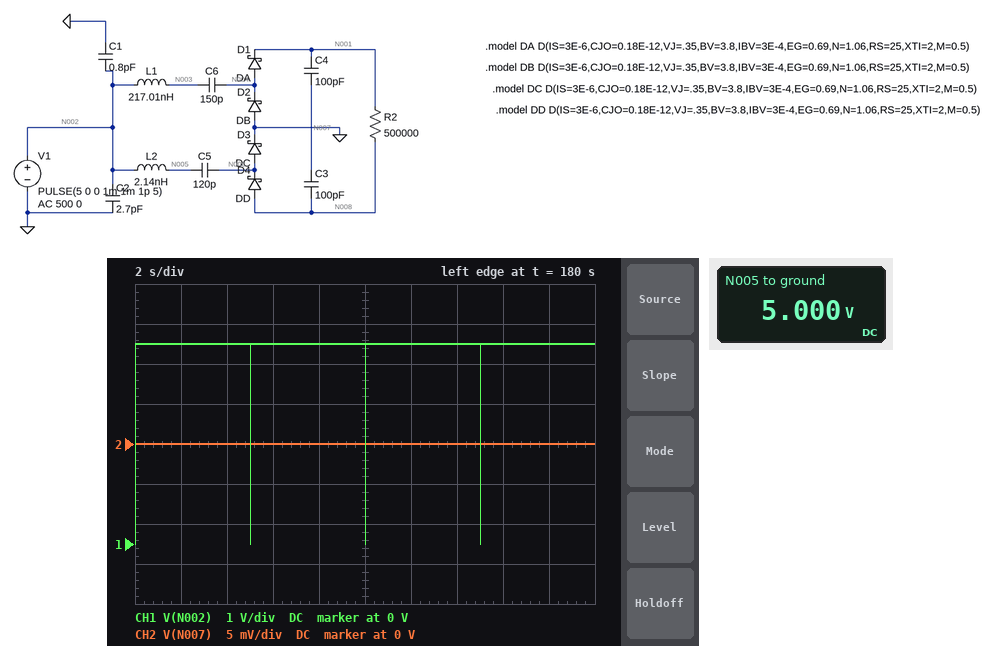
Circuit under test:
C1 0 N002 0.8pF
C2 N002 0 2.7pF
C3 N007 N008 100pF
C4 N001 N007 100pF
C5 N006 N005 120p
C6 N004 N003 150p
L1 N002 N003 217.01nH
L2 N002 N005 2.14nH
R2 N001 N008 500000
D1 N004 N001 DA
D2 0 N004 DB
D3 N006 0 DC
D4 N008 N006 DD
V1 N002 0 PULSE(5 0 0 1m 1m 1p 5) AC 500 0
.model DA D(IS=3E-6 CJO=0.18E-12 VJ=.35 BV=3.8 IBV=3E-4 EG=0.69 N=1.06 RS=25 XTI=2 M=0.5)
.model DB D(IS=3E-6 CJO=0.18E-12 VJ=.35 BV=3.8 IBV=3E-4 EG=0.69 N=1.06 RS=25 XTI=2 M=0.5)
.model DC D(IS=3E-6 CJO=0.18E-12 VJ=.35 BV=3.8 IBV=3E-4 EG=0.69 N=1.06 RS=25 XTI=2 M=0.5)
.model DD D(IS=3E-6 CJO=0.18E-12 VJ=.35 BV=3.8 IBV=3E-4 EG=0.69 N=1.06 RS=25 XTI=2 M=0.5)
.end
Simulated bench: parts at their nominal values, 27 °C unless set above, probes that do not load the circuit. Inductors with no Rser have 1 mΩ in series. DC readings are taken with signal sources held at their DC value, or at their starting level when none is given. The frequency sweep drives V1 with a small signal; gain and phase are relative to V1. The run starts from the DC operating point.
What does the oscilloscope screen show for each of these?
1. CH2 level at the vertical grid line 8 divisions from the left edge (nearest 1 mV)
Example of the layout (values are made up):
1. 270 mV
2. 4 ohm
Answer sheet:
1. 0 V
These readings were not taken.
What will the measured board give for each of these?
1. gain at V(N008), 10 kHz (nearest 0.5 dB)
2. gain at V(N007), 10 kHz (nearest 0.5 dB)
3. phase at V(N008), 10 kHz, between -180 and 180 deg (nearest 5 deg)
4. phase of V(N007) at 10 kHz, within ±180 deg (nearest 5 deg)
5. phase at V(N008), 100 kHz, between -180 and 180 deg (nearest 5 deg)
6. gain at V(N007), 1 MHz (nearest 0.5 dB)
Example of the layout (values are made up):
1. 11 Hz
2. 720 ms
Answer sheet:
1. -23.0 dB
2. -22.0 dB
3. 85 deg
4. 85 deg
5. 55 deg
6. 0 dB
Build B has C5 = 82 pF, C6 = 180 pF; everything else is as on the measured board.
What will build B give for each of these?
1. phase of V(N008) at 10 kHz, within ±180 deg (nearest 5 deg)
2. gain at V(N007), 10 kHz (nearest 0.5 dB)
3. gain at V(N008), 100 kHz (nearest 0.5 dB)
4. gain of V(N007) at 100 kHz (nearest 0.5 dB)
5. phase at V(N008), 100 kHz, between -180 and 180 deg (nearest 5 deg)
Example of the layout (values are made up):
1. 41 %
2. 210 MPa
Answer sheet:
1. 90 deg
2. -22.5 dB
3. -5.5 dB
4. -5.0 dB
5. 65 deg
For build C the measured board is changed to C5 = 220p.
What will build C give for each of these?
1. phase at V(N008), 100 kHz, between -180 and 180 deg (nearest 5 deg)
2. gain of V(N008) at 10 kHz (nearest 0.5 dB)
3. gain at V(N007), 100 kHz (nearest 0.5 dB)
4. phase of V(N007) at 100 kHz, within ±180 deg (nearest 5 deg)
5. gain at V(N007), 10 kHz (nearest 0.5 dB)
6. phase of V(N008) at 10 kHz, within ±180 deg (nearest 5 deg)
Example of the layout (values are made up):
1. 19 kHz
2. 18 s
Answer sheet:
1. 40 deg
2. -18.0 dB
3. -3.0 dB
4. 45 deg
5. -19.5 dB
6. 80 deg
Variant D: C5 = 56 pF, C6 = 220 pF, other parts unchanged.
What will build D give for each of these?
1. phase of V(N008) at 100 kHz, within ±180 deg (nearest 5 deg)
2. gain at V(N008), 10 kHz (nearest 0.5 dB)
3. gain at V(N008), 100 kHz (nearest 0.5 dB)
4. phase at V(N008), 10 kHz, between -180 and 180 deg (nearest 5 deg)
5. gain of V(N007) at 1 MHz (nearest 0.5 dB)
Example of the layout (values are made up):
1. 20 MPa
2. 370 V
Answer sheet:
1. 70 deg
2. -28.5 dB
3. -6.0 dB
4. 95 deg
5. -0.5 dB
